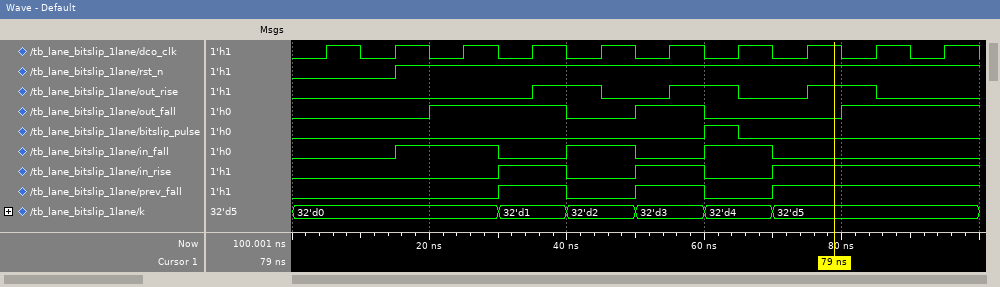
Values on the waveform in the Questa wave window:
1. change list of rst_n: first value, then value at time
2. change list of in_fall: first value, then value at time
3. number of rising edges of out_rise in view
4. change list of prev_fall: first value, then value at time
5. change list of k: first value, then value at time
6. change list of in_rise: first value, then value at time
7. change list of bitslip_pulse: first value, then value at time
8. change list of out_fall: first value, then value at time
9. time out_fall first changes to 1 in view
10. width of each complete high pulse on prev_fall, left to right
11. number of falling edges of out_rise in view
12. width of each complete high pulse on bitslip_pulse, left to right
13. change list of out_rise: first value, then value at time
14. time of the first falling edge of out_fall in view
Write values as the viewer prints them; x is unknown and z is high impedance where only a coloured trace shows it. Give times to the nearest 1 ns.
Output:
0, 1 at 15 ns
0, 1 at 15 ns, 0 at 30 ns, 1 at 40 ns, 0 at 50 ns, 1 at 60 ns, 0 at 70 ns
3
0, 1 at 30 ns, 0 at 40 ns, 1 at 50 ns, 0 at 60 ns, 1 at 70 ns
32'd0, 32'd1 at 30 ns, 32'd2 at 40 ns, 32'd3 at 50 ns, 32'd4 at 60 ns, 32'd5 at 70 ns
0, 1 at 30 ns, 0 at 40 ns, 1 at 50 ns, 0 at 60 ns, 1 at 70 ns
0, 1 at 60 ns, 0 at 65 ns
0, 1 at 20 ns, 0 at 40 ns, 1 at 50 ns, 0 at 60 ns, 1 at 80 ns
20 ns
10 ns, 10 ns
3
5 ns
0, 1 at 35 ns, 0 at 45 ns, 1 at 55 ns, 0 at 65 ns, 1 at 75 ns, 0 at 85 ns
40 ns
